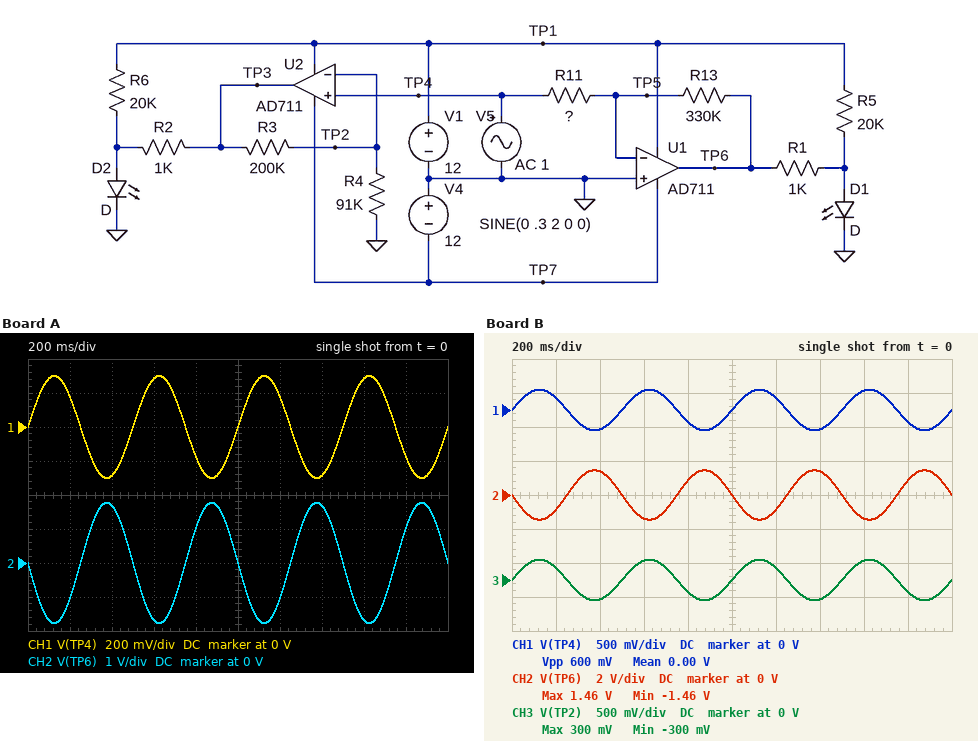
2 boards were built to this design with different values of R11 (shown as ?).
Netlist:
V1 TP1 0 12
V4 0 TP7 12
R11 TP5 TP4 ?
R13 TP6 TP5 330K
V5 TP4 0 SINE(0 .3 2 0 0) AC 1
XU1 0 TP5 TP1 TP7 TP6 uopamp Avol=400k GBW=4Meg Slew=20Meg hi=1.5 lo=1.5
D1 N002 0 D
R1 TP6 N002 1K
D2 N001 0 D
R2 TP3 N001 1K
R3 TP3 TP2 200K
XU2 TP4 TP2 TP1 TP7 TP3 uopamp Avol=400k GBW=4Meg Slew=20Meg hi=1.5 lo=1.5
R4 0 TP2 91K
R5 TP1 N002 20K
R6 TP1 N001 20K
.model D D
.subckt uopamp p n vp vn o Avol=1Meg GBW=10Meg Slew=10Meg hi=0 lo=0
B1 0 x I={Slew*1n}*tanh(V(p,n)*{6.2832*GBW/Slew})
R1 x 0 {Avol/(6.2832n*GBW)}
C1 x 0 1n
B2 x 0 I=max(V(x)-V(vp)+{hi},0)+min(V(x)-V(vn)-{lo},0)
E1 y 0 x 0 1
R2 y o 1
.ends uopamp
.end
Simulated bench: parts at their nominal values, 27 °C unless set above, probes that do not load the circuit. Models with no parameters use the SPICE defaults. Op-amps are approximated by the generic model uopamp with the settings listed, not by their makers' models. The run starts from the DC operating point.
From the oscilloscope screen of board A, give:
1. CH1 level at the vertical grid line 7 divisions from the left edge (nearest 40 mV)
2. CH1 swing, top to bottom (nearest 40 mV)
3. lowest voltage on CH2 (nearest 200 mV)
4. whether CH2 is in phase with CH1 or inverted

-280 mV
600 mV
-1.8 V
inverted
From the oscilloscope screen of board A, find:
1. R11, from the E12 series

56 kΩ
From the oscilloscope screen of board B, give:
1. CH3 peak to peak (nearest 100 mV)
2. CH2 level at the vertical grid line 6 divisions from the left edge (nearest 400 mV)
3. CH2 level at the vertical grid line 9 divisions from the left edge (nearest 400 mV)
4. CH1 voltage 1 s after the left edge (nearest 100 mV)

600 mV
-800 mV
800 mV
0 V
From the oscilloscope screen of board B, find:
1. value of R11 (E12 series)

68 kΩ
